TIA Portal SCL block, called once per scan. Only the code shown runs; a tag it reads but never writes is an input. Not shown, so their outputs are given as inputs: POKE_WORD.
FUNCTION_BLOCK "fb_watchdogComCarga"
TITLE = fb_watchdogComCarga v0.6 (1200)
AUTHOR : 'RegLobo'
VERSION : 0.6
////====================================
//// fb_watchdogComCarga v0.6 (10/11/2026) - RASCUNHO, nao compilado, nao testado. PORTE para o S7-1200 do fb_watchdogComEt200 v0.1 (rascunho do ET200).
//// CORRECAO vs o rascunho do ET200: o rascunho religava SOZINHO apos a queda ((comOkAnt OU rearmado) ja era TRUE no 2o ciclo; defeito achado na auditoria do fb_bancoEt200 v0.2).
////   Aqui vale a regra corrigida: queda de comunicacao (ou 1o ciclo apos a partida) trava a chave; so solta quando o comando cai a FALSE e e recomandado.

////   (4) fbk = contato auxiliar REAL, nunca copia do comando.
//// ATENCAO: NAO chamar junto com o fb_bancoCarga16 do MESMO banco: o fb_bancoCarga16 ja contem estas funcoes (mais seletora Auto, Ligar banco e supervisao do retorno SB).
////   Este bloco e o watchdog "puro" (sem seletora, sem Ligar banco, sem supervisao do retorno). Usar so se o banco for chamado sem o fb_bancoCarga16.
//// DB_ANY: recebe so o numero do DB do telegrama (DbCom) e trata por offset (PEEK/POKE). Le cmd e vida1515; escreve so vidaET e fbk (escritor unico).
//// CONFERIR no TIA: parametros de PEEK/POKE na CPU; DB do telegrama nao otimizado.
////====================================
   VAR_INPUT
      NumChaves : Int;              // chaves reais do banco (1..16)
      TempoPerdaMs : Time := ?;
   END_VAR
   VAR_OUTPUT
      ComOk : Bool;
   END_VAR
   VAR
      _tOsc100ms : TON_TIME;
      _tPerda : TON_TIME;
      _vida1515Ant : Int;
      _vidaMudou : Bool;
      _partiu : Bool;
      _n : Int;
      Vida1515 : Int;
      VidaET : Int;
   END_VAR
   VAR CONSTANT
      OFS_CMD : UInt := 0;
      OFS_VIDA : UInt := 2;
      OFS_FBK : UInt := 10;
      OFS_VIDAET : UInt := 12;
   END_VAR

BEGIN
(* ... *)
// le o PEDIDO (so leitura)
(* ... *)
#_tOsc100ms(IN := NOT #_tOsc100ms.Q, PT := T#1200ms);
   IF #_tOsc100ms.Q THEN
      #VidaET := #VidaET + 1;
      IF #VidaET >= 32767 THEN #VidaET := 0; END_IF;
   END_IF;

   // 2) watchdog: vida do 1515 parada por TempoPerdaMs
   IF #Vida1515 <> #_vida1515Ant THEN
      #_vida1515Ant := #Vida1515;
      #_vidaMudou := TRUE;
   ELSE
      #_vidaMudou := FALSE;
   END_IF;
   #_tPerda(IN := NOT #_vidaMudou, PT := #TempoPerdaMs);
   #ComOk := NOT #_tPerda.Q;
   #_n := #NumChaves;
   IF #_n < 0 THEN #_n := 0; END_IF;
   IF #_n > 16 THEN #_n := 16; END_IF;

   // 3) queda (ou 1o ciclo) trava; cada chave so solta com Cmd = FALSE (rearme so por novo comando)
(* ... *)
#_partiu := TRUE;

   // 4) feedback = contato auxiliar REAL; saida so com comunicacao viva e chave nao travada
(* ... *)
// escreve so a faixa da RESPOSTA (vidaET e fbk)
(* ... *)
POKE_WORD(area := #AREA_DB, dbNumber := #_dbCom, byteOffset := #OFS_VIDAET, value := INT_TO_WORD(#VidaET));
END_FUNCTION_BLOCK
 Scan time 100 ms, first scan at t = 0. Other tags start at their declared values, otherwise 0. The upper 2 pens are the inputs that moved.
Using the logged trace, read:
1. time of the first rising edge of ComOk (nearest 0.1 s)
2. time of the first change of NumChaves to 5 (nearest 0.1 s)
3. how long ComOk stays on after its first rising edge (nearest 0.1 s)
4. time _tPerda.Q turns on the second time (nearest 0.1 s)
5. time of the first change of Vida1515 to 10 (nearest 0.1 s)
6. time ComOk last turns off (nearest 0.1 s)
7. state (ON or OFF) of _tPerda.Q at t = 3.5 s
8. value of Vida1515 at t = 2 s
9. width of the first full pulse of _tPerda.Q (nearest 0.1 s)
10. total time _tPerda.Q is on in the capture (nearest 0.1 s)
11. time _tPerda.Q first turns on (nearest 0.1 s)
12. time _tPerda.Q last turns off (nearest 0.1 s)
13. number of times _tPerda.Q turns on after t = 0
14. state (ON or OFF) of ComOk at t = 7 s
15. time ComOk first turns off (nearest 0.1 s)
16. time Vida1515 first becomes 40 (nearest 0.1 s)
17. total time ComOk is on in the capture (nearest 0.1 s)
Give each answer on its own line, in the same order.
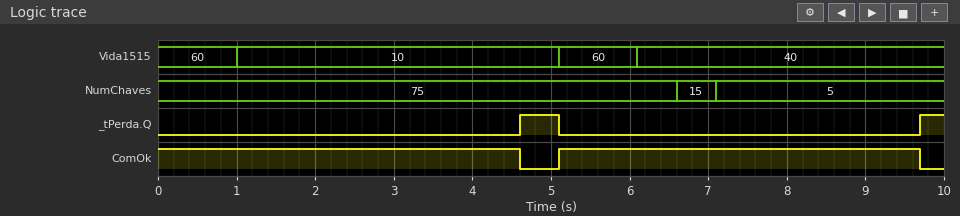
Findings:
5.1 s
7.1 s
4.6 s
9.7 s
1.0 s
9.7 s
OFF
10
0.5 s
0.8 s
4.6 s
5.1 s
2
ON
4.6 s
6.1 s
9.2 s
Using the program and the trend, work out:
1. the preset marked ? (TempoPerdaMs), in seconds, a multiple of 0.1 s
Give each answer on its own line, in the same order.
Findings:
3.5 s
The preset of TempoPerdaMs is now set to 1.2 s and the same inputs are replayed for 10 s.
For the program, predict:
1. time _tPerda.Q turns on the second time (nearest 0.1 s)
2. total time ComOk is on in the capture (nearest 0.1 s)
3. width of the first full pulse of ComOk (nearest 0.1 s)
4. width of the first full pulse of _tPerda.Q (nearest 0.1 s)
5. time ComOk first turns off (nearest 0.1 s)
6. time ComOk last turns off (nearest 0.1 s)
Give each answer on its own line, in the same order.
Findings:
7.4 s
4.6 s
2.3 s
2.8 s
2.3 s
7.4 s
